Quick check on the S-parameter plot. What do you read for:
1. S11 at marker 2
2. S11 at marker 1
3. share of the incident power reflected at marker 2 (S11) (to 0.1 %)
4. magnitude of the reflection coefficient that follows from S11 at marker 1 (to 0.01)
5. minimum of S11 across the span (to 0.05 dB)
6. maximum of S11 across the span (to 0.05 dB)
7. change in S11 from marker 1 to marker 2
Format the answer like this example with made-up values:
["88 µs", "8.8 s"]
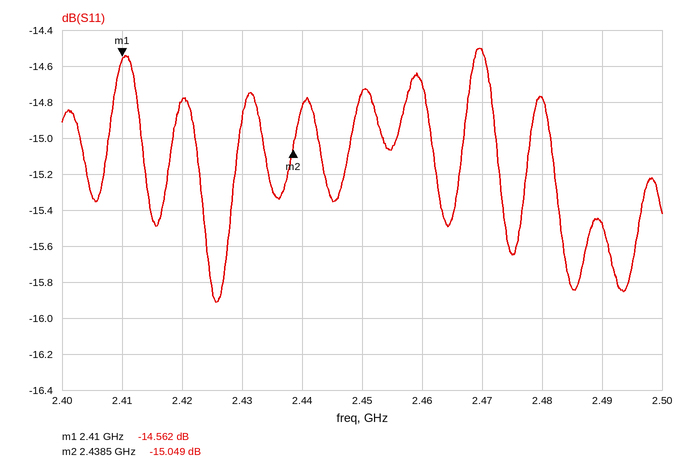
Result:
["-15.049 dB", "-14.562 dB", "3.1 %", "0.19", "-15.90 dB", "-14.50 dB", "-0.487 dB"]
